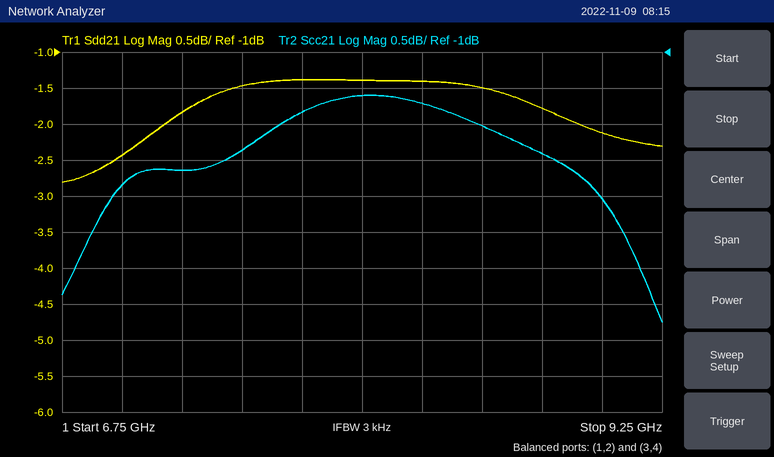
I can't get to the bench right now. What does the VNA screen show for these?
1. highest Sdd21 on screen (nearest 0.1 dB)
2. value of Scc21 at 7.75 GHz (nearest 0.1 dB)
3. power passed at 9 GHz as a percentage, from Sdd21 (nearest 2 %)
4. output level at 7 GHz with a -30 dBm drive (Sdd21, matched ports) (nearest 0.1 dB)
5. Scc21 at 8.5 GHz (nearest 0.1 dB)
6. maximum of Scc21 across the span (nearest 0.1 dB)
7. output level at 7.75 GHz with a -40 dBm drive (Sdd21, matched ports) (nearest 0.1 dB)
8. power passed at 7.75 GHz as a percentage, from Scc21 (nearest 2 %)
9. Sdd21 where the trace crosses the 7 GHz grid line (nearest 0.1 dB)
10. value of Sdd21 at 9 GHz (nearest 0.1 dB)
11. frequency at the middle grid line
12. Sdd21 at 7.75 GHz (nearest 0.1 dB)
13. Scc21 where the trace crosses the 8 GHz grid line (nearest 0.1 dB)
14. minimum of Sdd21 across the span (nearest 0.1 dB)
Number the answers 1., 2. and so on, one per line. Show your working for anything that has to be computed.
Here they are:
1. -1.4 dB
2. -1.8 dB
3. 10^(-2.1/10) ≈ 62 %
4. -30 dBm + (-2.4 dB) = -32.4 dBm
5. -2.0 dB
6. -1.6 dB
7. -40 dBm + (-1.4 dB) = -41.4 dBm
8. 10^(-1.8/10) ≈ 66 %
9. -2.4 dB
10. -2.1 dB
11. 8 GHz
12. -1.4 dB
13. -1.6 dB
14. -2.8 dB
